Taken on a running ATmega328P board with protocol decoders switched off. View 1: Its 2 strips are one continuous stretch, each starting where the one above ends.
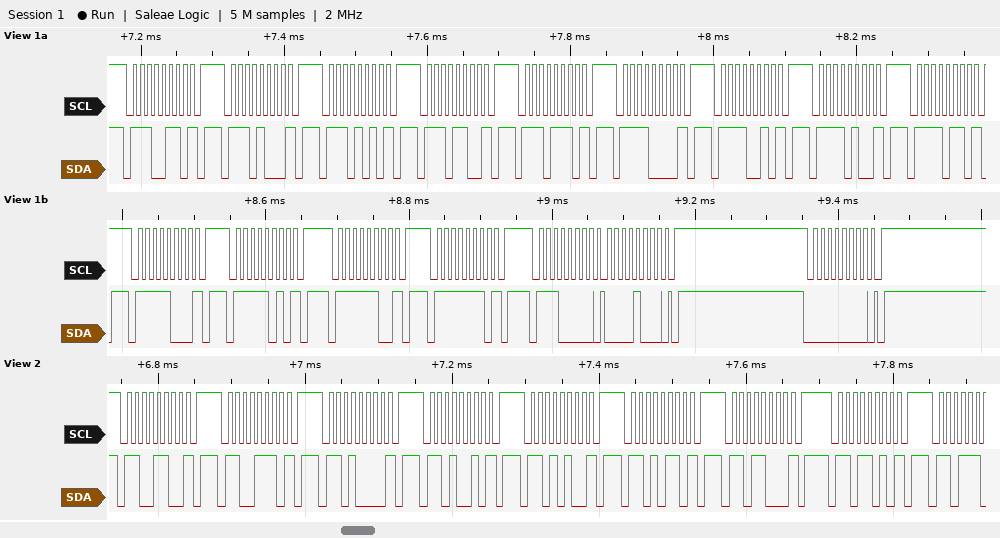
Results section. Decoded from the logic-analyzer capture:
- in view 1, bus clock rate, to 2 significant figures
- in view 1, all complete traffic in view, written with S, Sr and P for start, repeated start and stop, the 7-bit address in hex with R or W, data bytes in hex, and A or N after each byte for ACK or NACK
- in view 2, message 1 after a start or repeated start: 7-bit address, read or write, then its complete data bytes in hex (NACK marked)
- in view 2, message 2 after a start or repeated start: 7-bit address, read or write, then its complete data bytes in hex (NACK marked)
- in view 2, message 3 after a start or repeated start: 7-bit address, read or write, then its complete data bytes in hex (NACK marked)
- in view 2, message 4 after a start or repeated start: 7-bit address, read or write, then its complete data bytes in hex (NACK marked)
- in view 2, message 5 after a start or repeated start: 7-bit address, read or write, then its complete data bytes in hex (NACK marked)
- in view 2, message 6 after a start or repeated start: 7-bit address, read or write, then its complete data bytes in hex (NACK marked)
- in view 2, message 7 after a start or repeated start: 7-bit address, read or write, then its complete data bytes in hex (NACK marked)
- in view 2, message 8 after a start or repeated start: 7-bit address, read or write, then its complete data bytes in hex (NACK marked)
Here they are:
100 kHz
S 73W N P S 74W N P S 75W N P S 76W N P S 77W N P S 78W N P S 79W N P S 7AW N P S 7BW N P S 7CW N P S 7DW N P S 7EW N P S 7FW N P S 70W A 08 A P S 00W A P
0x66 write NACK
0x67 write NACK
0x68 write NACK
0x69 write NACK
0x6A write NACK
0x6B write NACK
0x6C write NACK
0x6D write NACK
